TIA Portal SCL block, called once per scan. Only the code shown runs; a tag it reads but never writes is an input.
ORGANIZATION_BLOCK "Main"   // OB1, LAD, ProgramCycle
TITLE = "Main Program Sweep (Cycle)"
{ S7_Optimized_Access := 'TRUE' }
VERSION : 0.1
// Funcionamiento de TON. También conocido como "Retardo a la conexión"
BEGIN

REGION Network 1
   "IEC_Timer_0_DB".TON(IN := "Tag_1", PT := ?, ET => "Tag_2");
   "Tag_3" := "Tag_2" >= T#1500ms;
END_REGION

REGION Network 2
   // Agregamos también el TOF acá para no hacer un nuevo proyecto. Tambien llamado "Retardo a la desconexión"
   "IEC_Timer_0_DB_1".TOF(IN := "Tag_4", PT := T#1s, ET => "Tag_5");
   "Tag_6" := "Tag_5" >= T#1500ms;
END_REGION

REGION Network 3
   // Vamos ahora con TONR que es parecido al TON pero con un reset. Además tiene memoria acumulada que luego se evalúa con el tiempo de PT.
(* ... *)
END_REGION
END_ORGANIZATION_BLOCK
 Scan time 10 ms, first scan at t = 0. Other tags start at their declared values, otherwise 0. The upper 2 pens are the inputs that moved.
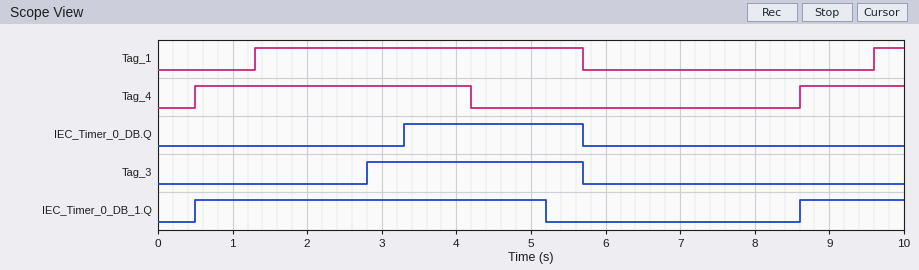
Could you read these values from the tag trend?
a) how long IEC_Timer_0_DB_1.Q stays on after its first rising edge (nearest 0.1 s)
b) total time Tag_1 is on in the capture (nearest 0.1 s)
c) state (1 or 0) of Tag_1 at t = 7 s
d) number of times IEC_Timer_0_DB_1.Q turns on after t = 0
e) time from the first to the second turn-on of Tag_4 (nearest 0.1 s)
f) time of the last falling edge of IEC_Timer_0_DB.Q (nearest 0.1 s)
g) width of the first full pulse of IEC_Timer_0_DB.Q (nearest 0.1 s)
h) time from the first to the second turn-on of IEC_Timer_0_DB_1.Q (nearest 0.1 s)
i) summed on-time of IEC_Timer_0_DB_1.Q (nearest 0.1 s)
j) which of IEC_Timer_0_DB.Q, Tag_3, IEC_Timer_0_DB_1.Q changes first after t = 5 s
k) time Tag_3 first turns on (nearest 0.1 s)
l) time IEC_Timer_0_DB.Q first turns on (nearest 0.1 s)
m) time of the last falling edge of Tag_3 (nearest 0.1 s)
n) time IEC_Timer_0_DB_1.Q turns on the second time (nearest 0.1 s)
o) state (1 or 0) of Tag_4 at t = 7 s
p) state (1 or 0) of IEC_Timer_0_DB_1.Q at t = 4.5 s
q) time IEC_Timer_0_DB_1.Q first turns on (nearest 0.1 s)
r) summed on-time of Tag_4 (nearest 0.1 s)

4.7 s
4.8 s
0
2
8.1 s
5.7 s
2.4 s
8.1 s
6.1 s
IEC_Timer_0_DB_1.Q
2.8 s
3.3 s
5.7 s
8.6 s
0
1
0.5 s
5.1 s
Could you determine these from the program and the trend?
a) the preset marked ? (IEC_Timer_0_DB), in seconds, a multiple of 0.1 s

2.0 s
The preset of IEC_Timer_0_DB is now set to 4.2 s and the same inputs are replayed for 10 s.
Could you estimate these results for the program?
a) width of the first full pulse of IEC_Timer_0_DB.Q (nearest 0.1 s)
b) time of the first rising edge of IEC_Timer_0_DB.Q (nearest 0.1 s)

0.2 s
5.5 s
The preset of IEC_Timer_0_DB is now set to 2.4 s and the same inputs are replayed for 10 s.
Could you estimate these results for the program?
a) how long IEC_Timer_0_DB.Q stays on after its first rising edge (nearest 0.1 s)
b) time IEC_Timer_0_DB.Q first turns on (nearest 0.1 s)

2.0 s
3.7 s
